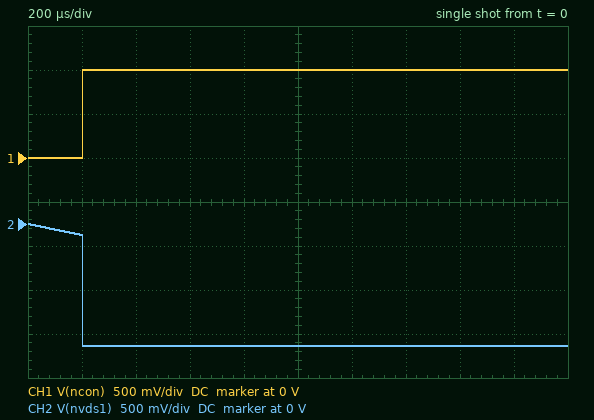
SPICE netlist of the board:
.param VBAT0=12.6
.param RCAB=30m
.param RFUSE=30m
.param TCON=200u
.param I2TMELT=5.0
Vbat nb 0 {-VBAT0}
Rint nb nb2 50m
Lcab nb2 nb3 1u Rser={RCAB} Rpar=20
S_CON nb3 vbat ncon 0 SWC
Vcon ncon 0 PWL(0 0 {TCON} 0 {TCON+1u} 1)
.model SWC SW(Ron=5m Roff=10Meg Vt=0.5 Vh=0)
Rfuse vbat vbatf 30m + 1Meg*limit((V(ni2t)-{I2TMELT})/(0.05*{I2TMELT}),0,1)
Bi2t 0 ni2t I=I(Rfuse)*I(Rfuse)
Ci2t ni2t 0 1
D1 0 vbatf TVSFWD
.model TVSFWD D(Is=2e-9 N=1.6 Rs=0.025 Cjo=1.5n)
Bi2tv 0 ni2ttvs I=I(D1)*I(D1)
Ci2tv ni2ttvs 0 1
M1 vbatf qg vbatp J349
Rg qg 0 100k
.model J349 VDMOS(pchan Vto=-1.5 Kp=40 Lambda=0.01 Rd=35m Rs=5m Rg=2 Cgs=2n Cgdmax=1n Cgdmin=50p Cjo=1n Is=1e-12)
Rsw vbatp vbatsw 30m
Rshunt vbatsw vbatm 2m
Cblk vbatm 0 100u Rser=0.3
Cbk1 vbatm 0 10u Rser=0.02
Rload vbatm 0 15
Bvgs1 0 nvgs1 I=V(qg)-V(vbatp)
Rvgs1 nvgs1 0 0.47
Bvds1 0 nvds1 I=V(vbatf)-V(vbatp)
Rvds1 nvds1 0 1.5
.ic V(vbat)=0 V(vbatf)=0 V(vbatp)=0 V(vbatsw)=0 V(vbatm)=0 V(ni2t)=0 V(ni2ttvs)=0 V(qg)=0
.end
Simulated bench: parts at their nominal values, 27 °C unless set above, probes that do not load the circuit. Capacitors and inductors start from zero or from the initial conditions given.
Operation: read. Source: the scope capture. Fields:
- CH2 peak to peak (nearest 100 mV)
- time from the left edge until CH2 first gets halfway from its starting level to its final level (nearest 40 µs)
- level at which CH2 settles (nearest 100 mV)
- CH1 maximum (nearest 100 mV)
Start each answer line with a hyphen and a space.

- 1.4 V
- 200 µs
- -1.4 V
- 1.0 V
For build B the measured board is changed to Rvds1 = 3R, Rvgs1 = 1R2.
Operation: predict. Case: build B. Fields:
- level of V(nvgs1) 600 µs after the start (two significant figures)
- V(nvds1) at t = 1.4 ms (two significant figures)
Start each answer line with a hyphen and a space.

- -40 mV
- -2.8 V
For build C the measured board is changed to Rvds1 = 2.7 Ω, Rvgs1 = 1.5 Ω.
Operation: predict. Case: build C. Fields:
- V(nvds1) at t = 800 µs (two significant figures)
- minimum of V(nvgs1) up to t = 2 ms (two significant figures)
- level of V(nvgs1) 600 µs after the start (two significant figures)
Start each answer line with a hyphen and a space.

- -2.5 V
- -270 mV
- -50 mV
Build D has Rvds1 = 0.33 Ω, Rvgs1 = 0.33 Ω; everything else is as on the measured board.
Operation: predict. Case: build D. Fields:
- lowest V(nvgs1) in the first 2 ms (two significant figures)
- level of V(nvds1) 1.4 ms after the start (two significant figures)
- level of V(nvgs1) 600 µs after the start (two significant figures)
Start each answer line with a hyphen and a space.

- -59 mV
- -300 mV
- -11 mV
